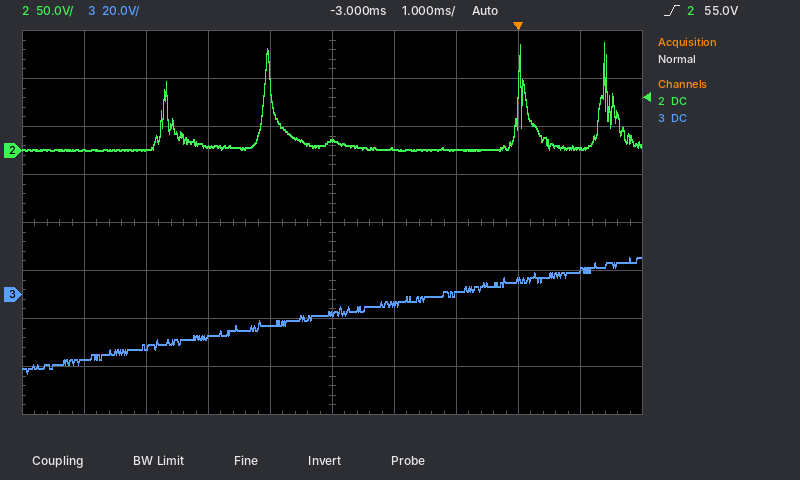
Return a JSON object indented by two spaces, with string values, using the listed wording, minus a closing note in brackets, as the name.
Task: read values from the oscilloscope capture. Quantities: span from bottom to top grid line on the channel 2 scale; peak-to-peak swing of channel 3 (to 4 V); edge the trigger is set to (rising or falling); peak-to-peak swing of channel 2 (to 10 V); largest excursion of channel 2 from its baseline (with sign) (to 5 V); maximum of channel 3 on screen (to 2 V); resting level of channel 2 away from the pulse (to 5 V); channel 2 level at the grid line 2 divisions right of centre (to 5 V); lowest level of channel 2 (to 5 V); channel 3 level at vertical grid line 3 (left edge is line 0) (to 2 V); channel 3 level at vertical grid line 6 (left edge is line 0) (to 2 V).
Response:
{
  "span from bottom to top grid line on the channel 2 scale": "400 V",
  "peak-to-peak swing of channel 3": "48 V",
  "edge the trigger is set to": "rising",
  "peak-to-peak swing of channel 2": "110 V",
  "largest excursion of channel 2 from its baseline (with sign)": "+110 V",
  "maximum of channel 3 on screen": "16 V",
  "resting level of channel 2 away from the pulse": "0 V",
  "channel 2 level at the grid line 2 divisions right of centre": "0 V",
  "lowest level of channel 2": "0 V",
  "channel 3 level at vertical grid line 3 (left edge is line 0)": "-18 V",
  "channel 3 level at vertical grid line 6 (left edge is line 0)": "-4 V"
}
